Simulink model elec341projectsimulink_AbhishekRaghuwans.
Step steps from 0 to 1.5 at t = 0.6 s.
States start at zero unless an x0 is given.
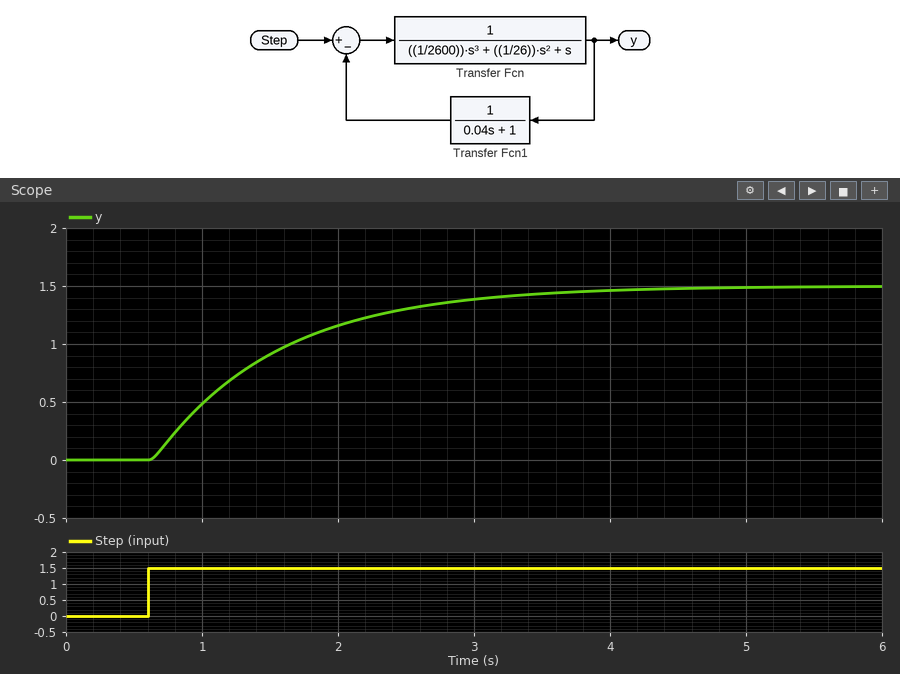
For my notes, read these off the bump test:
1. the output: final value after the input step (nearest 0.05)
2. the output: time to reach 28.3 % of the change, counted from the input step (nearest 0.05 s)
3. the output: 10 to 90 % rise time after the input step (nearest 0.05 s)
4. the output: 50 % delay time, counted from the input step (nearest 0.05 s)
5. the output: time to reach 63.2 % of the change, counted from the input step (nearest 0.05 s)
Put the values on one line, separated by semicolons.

1.50; 0.35 s; 2.00 s; 0.70 s; 0.95 s
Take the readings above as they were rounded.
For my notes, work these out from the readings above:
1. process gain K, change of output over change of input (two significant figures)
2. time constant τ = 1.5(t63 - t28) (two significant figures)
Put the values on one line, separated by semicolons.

1.0; 0.90 s
